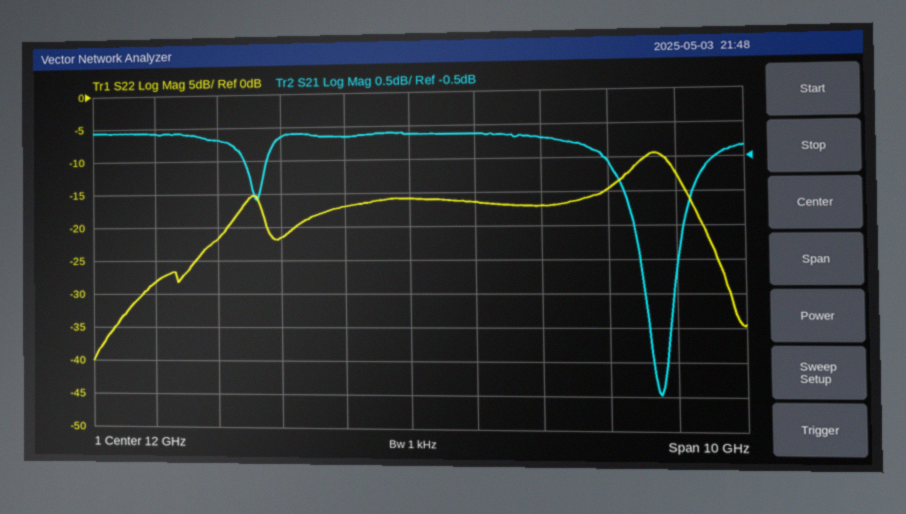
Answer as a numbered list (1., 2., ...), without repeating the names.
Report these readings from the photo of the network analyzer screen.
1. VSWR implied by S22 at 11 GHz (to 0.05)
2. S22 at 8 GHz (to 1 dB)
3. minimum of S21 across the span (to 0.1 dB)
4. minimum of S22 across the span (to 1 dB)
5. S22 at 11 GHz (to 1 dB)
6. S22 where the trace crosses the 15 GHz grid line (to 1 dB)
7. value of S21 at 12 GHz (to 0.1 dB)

1. 1.35
2. -28 dB
3. -4.0 dB
4. -40 dB
5. -17 dB
6. -15 dB
7. -0.1 dB
